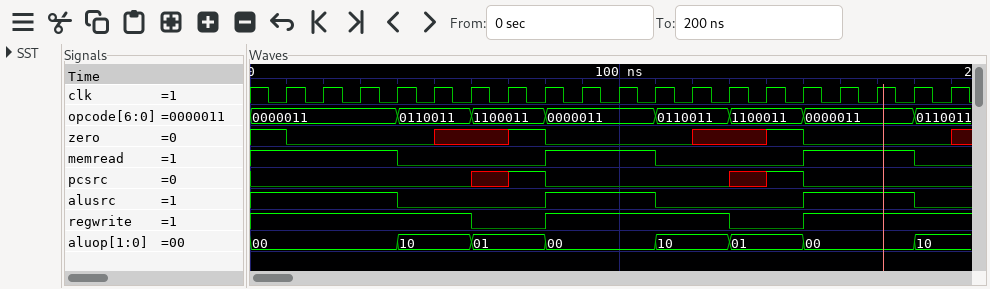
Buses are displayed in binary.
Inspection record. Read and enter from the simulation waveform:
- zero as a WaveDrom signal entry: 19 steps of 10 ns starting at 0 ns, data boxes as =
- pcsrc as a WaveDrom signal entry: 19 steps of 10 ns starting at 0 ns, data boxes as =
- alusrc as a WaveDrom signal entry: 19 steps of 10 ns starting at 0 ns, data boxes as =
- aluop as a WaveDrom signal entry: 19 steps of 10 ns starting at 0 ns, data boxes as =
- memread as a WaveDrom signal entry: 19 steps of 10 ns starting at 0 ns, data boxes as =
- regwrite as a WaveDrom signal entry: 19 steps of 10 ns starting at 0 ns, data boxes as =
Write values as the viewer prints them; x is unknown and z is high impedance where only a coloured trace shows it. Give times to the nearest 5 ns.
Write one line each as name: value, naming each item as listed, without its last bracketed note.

zero as a WaveDrom signal entry: 19 steps of 10 ns starting at 0 ns, data boxes as =: {name: 'zero', wave: '10...x.10...x.10...'}
pcsrc as a WaveDrom signal entry: 19 steps of 10 ns starting at 0 ns, data boxes as =: {name: 'pcsrc', wave: '0.....x10....x10...'}
alusrc as a WaveDrom signal entry: 19 steps of 10 ns starting at 0 ns, data boxes as =: {name: 'alusrc', wave: '1...0...1..0...1..0'}
aluop as a WaveDrom signal entry: 19 steps of 10 ns starting at 0 ns, data boxes as =: {name: 'aluop', wave: '=...=.=.=..=.=.=..=', data: '00 10 01 00 10 01 00 10'}
memread as a WaveDrom signal entry: 19 steps of 10 ns starting at 0 ns, data boxes as =: {name: 'memread', wave: '1...0...1..0...1..0'}
regwrite as a WaveDrom signal entry: 19 steps of 10 ns starting at 0 ns, data boxes as =: {name: 'regwrite', wave: '1.....0.1....0.1...'}
